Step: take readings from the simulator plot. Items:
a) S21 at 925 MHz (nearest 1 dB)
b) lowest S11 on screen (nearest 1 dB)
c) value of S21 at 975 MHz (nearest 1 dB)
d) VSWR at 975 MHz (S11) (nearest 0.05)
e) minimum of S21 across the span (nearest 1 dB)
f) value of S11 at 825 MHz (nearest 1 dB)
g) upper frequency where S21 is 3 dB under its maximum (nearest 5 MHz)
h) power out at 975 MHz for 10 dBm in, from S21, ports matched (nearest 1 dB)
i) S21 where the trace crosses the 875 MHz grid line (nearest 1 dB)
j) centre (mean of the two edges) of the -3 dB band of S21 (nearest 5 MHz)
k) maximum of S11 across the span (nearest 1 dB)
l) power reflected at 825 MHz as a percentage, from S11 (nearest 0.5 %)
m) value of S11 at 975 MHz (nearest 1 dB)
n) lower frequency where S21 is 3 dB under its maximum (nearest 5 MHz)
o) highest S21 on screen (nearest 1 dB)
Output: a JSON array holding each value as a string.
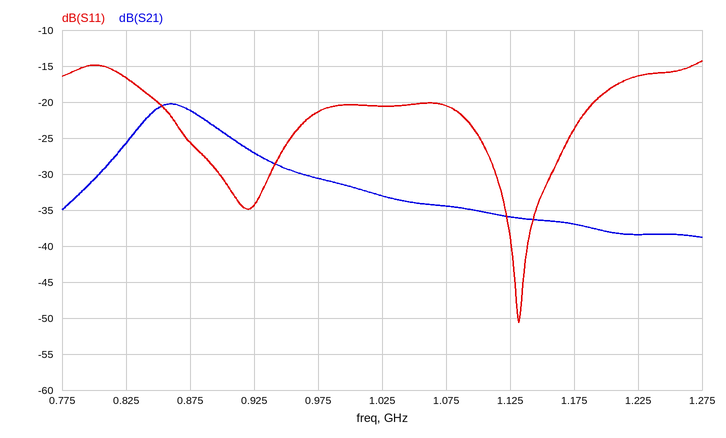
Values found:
["-27 dB", "-51 dB", "-31 dB", "1.20", "-39 dB", "-17 dB", "895 MHz", "-21 dBm", "-21 dB", "865 MHz", "-14 dB", "2.0 %", "-21 dB", "835 MHz", "-20 dB"]
